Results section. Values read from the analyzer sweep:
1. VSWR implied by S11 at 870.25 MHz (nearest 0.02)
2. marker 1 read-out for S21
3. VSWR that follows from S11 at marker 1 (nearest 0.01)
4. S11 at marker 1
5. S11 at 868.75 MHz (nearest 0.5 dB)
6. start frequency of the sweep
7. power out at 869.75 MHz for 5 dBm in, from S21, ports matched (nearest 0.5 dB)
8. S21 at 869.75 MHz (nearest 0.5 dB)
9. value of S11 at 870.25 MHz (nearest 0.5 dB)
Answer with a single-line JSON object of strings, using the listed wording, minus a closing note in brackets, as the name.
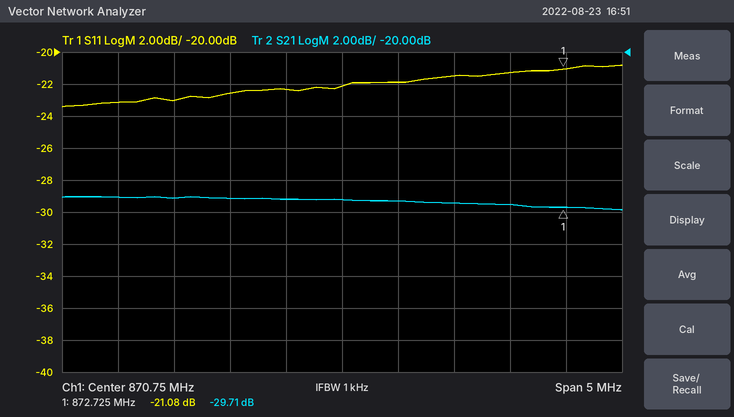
{"VSWR implied by S11 at 870.25 MHz": "1.16", "marker 1 read-out for S21": "-29.71 dB", "VSWR that follows from S11 at marker 1": "1.19", "S11 at marker 1": "-21.08 dB", "S11 at 868.75 MHz": "-23.0 dB", "start frequency of the sweep": "868.25 MHz", "power out at 869.75 MHz for 5 dBm in, from S21, ports matched": "-24.0 dBm", "S21 at 869.75 MHz": "-29.0 dB", "value of S11 at 870.25 MHz": "-22.5 dB"}
